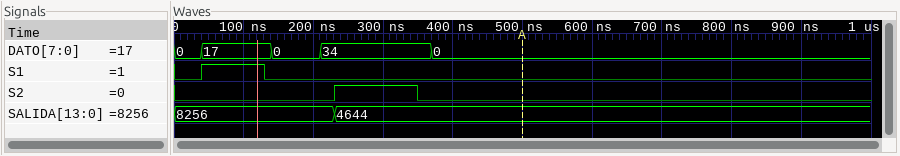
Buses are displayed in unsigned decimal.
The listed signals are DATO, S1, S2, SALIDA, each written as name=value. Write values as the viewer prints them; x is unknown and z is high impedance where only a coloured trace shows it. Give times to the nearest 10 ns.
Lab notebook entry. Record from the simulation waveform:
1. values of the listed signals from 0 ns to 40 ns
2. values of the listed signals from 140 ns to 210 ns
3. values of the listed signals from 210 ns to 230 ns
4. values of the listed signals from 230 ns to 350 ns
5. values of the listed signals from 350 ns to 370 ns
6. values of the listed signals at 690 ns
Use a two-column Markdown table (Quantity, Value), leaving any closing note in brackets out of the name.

| Quantity | Value |
|---|---|
| values of the listed signals from 0 ns to 40 ns | DATO=0, S1=0, S2=0, SALIDA=8256 |
| values of the listed signals from 140 ns to 210 ns | DATO=0, S1=0, S2=0, SALIDA=8256 |
| values of the listed signals from 210 ns to 230 ns | DATO=34, S1=0, S2=0, SALIDA=8256 |
| values of the listed signals from 230 ns to 350 ns | DATO=34, S1=0, S2=1, SALIDA=4644 |
| values of the listed signals from 350 ns to 370 ns | DATO=34, S1=0, S2=0, SALIDA=4644 |
| values of the listed signals at 690 ns | DATO=0, S1=0, S2=0, SALIDA=4644 |
